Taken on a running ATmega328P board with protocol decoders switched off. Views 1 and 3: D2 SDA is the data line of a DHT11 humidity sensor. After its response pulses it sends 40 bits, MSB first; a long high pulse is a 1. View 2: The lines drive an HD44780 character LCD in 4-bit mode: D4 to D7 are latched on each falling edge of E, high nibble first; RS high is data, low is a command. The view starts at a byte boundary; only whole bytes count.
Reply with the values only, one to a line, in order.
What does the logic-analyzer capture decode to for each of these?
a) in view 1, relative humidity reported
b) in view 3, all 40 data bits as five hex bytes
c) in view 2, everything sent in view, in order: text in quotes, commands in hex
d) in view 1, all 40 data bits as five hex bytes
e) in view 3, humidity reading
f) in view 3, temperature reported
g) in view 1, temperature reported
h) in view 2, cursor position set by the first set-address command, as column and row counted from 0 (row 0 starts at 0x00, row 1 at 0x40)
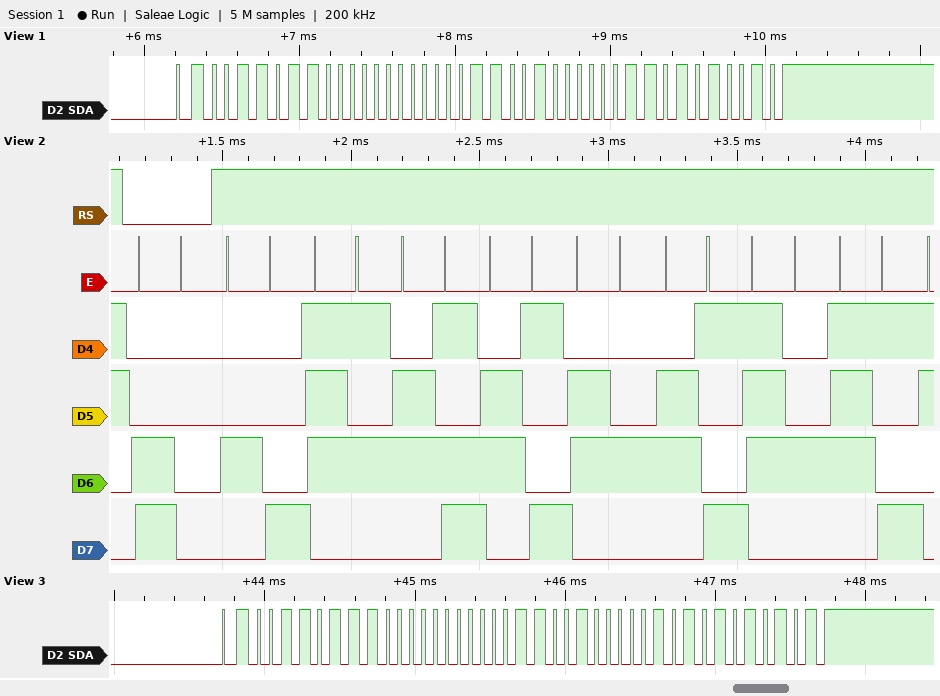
54 %
37 00 19 05 55
0xC0 "Humidity"
36 00 19 03 52
55 %
25.5 °C
25.3 °C
column 0, row 1
